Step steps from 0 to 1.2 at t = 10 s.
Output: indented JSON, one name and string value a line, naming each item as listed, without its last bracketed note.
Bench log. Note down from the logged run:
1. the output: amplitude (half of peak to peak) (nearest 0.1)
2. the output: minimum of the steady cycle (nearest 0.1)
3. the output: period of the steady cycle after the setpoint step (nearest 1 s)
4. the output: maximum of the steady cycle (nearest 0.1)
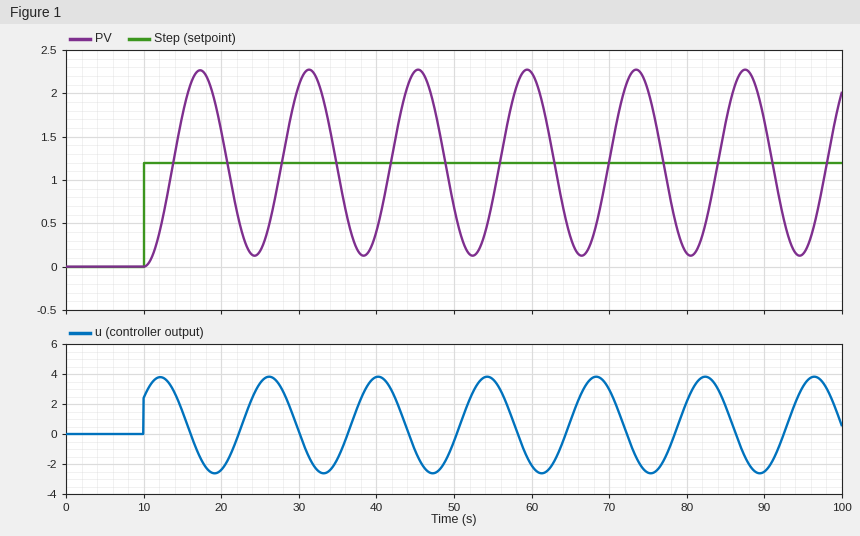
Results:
{
  "the output: amplitude (half of peak to peak)": "1.1",
  "the output: minimum of the steady cycle": "0.1",
  "the output: period of the steady cycle after the setpoint step": "14 s",
  "the output: maximum of the steady cycle": "2.3"
}
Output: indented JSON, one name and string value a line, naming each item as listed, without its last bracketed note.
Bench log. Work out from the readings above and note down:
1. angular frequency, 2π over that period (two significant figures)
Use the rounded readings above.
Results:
{
  "angular frequency, 2π over that period": "0.45 rad/s"
}
